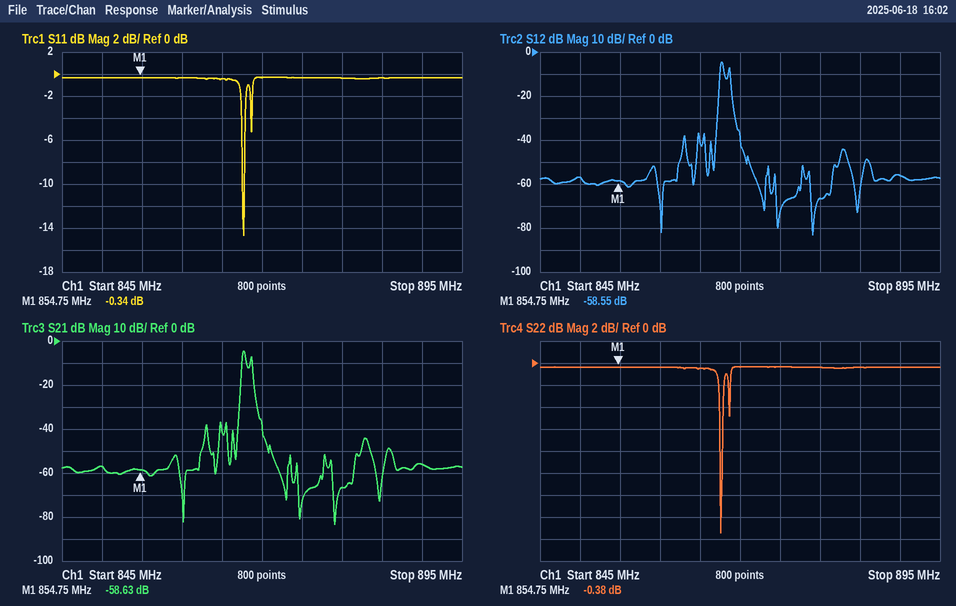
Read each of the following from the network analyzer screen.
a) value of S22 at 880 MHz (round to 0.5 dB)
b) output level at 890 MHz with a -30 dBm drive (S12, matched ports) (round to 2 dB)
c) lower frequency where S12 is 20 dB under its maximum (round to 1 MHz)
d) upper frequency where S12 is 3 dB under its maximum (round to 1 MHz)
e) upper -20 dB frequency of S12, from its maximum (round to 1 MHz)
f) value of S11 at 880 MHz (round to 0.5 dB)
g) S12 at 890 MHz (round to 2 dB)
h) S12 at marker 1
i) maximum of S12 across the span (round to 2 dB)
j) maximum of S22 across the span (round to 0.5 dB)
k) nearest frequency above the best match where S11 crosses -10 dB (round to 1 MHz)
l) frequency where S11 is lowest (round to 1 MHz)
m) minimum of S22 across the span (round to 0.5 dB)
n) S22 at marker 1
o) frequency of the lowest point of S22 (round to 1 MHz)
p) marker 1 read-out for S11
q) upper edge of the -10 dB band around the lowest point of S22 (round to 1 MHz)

-0.5 dB
-86 dBm
867 MHz
868 MHz
869 MHz
-0.5 dB
-56 dB
-58.55 dB
-4 dB
-0.5 dB
868 MHz
868 MHz
-15.5 dB
-0.38 dB
868 MHz
-0.34 dB
868 MHz
